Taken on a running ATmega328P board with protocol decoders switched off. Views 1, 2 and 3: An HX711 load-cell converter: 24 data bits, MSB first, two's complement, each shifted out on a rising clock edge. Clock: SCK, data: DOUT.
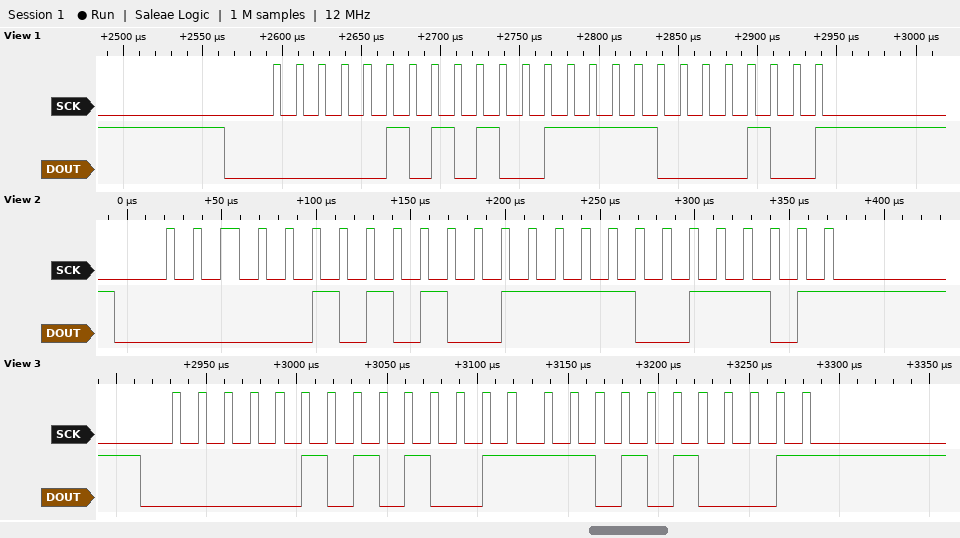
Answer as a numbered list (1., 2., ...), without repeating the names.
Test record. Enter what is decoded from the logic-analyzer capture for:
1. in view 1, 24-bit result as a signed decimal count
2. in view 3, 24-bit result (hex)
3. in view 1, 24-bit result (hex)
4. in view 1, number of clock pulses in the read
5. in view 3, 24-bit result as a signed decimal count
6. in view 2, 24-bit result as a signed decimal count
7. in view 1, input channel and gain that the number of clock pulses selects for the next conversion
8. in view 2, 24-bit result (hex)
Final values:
1. 348036
2. 0x054F51
3. 0x054F84
4. 25
5. 347985
6. 348061
7. channel A, gain 128
8. 0x054F9D
